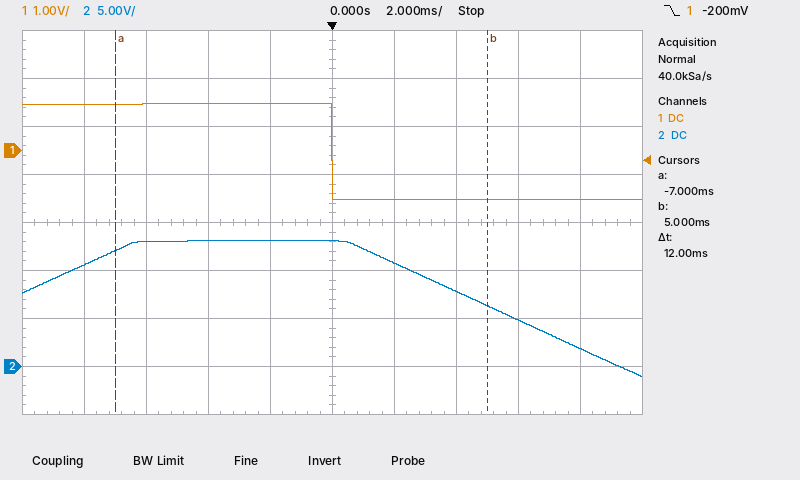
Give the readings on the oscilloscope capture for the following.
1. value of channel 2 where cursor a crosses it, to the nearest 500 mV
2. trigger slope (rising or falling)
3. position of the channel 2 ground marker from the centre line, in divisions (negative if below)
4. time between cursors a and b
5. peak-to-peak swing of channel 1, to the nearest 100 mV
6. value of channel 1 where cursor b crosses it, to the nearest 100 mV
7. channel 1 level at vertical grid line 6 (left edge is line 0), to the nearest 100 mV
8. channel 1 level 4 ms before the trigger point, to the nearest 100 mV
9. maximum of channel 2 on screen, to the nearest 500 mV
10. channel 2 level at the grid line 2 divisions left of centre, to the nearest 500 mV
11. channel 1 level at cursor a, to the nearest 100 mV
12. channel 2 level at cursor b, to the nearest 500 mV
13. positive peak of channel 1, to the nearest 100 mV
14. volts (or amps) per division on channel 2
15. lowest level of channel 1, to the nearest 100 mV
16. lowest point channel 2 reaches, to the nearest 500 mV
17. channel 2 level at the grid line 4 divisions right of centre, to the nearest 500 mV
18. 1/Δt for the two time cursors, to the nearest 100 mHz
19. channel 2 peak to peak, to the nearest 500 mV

12.0 V
falling
-3.0 div
12 ms
2.0 V
-1.0 V
-1.0 V
1.0 V
13.0 V
13.0 V
1.0 V
6.5 V
1.0 V
5 V
-1.0 V
-1.0 V
2.0 V
83.3 Hz
14.0 V
